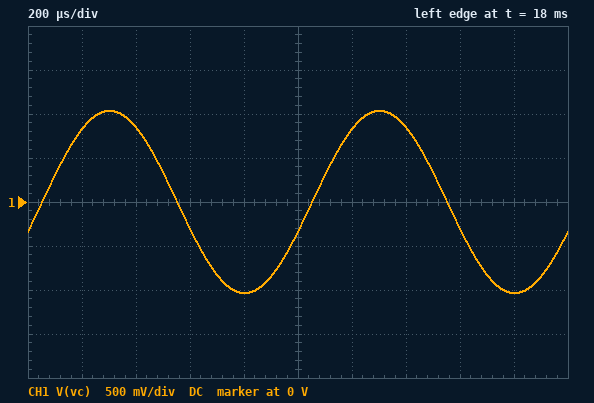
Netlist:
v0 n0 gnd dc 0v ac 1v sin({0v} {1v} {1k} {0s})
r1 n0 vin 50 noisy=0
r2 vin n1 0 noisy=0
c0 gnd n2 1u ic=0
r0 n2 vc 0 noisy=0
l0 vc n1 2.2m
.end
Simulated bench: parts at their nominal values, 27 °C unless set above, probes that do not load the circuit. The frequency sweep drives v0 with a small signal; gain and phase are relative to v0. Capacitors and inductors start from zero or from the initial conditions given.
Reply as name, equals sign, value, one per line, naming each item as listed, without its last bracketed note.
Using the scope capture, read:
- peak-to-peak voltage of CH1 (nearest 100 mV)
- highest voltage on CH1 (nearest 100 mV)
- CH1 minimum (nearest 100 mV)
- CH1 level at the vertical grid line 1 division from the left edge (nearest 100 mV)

peak-to-peak voltage of CH1 = 2.1 V
highest voltage on CH1 = 1.0 V
CH1 minimum = -1.0 V
CH1 level at the vertical grid line 1 division from the left edge = 800 mV
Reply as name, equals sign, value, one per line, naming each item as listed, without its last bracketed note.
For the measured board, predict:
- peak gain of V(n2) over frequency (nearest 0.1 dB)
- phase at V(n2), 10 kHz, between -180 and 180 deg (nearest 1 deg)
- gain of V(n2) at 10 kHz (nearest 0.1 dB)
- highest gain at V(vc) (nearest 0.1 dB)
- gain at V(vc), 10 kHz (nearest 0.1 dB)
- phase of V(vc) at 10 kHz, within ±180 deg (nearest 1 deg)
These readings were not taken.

peak gain of V(n2) over frequency = 0.9 dB
phase at V(n2), 10 kHz, between -180 and 180 deg = -158 deg
gain of V(n2) at 10 kHz = -18.4 dB
highest gain at V(vc) = 0.9 dB
gain at V(vc), 10 kHz = -18.4 dB
phase of V(vc) at 10 kHz, within ±180 deg = -158 deg
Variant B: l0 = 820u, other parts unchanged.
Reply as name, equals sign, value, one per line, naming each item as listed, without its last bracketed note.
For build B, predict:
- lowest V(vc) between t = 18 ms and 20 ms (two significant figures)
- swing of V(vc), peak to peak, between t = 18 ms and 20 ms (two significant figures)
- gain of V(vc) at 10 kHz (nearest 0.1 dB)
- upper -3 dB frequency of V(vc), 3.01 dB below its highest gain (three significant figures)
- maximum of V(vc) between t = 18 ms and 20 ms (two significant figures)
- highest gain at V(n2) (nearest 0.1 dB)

lowest V(vc) between t = 18 ms and 20 ms = -980 mV
swing of V(vc), peak to peak, between t = 18 ms and 20 ms = 2.0 V
gain of V(vc) at 10 kHz = -11.7 dB
upper -3 dB frequency of V(vc), 3.01 dB below its highest gain = 4.33 kHz
maximum of V(vc) between t = 18 ms and 20 ms = 980 mV
highest gain at V(n2) = 0 dB
